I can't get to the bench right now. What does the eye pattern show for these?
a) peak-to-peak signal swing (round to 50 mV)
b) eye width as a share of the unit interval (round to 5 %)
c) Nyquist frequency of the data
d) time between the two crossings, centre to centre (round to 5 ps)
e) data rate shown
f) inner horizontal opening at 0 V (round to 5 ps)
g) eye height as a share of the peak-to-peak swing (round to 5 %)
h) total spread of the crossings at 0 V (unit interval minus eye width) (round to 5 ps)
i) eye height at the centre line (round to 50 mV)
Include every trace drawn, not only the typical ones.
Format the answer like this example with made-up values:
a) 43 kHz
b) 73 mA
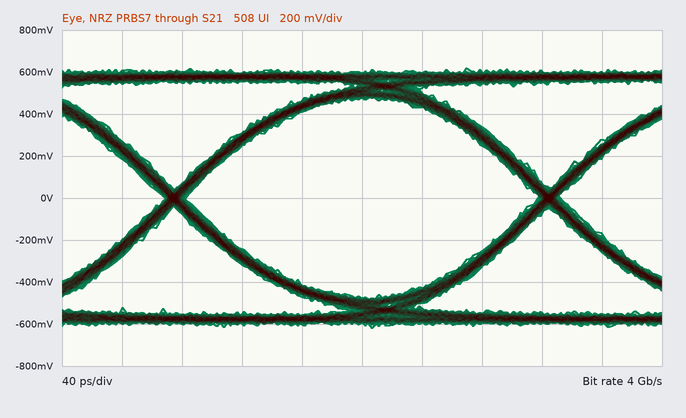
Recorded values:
a) 1.25 V
b) 95 %
c) 2 GHz
d) 250 ps
e) 4 Gb/s
f) 235 ps
g) 75 %
h) 15 ps
i) 950 mV
